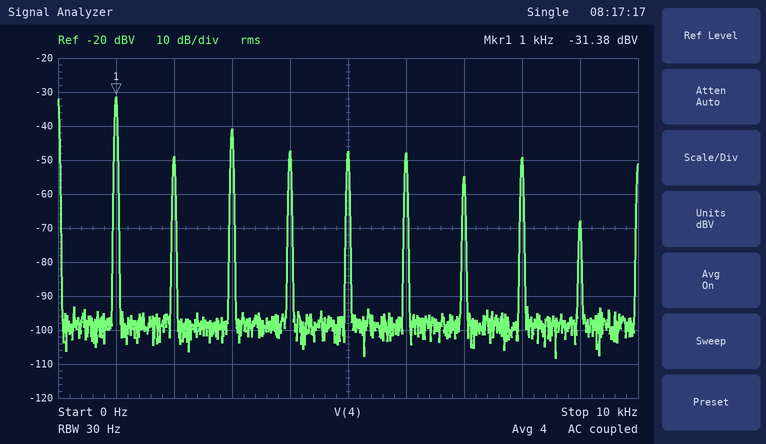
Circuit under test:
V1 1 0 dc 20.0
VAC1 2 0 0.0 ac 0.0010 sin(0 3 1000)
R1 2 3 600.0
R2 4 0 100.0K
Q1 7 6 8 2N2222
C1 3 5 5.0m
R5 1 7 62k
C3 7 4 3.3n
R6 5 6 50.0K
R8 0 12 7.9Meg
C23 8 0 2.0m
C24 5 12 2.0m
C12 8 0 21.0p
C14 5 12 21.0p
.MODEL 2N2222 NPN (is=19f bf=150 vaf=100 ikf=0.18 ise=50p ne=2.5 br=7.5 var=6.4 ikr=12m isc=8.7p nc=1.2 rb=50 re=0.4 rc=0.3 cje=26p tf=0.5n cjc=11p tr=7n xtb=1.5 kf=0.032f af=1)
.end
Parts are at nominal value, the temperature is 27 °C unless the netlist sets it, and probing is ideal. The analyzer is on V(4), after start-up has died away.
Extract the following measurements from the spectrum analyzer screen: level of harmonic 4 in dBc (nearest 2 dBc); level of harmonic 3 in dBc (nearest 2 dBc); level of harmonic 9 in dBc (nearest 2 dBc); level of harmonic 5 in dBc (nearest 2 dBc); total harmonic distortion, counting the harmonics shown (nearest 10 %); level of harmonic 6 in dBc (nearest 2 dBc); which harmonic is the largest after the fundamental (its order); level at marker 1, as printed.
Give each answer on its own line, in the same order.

-16 dBc
-10 dBc
-36 dBc
-16 dBc
50 %
-16 dBc
3
-31.38 dBV
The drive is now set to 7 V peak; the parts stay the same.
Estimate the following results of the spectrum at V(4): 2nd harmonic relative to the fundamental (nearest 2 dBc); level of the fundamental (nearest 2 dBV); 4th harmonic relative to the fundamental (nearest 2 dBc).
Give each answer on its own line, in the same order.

-24 dBc
-32 dBV
-24 dBc
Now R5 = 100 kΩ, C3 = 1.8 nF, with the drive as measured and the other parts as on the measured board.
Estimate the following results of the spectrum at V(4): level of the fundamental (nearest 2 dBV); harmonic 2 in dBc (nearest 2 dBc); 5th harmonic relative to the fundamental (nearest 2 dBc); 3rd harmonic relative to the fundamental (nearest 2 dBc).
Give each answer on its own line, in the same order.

-34 dBV
-20 dBc
-14 dBc
-8 dBc
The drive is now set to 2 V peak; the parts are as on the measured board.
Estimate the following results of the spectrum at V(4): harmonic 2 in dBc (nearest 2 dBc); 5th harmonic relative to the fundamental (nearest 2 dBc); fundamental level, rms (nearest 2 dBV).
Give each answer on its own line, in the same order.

-12 dBc
-22 dBc
-32 dBV
